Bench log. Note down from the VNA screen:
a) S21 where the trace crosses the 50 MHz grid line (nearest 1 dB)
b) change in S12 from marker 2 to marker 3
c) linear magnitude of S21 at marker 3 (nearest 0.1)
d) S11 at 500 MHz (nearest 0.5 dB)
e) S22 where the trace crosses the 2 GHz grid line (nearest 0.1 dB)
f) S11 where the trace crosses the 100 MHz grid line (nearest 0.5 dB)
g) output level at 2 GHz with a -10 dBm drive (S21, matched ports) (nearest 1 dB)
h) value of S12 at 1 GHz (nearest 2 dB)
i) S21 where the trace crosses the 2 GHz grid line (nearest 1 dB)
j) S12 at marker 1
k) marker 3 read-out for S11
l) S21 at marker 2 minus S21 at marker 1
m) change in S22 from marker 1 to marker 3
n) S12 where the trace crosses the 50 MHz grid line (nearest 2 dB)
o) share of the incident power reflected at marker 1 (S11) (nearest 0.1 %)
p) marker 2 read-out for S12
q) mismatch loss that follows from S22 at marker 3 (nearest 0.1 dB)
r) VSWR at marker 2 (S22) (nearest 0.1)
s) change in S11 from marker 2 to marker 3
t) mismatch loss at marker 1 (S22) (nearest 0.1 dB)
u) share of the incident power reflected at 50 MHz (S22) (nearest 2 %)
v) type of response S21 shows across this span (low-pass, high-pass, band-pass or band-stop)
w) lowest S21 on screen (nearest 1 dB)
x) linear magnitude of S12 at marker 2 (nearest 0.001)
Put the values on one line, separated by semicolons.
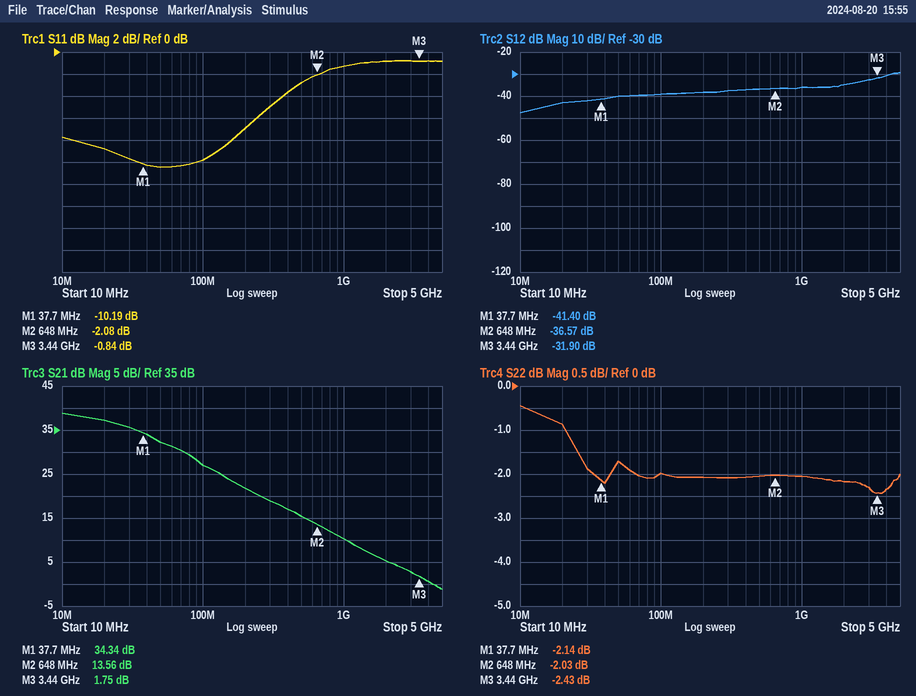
32 dB; 4.67 dB; 1.2; -3.0 dB; -2.2 dB; -10.0 dB; -5 dBm; -36 dB; 5 dB; -41.40 dB; -0.84 dB; -20.78 dB; -0.29 dB; -40 dB; 9.6 %; -36.57 dB; 3.7 dB; 8.6; 1.24 dB; 4.1 dB; 68 %; low-pass; -1 dB; 0.015
